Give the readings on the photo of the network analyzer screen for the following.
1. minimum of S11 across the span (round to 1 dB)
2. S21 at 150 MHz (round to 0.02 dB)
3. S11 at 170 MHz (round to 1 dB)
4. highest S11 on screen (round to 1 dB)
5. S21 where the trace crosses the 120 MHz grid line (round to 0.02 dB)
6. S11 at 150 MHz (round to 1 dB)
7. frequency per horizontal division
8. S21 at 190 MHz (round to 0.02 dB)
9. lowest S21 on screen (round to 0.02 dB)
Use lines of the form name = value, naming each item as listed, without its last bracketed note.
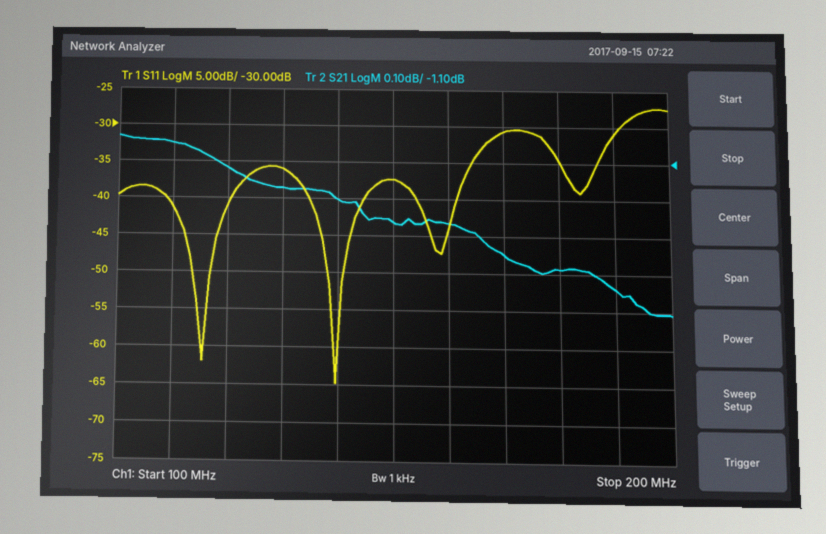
minimum of S11 across the span = -65 dB
S21 at 150 MHz = -1.26 dB
S11 at 170 MHz = -31 dB
highest S11 on screen = -27 dB
S21 where the trace crosses the 120 MHz grid line = -1.12 dB
S11 at 150 MHz = -37 dB
frequency per horizontal division = 10 MHz
S21 at 190 MHz = -1.44 dB
lowest S21 on screen = -1.50 dB
